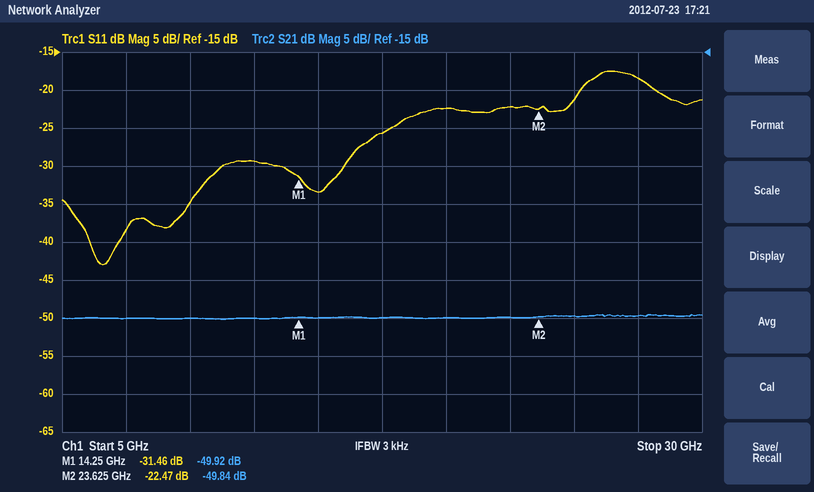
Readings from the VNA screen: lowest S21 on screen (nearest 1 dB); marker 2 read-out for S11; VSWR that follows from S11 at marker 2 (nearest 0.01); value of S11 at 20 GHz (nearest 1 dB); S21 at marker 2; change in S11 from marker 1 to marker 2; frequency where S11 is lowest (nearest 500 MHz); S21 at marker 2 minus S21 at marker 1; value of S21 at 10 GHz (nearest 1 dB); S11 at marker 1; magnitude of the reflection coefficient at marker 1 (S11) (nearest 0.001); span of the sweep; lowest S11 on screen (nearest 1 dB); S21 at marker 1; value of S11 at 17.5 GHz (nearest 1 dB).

-50 dB
-22.47 dB
1.16
-22 dB
-49.84 dB
8.99 dB
6.5 GHz
0.08 dB
-50 dB
-31.46 dB
0.027
25 GHz
-43 dB
-49.92 dB
-26 dB
